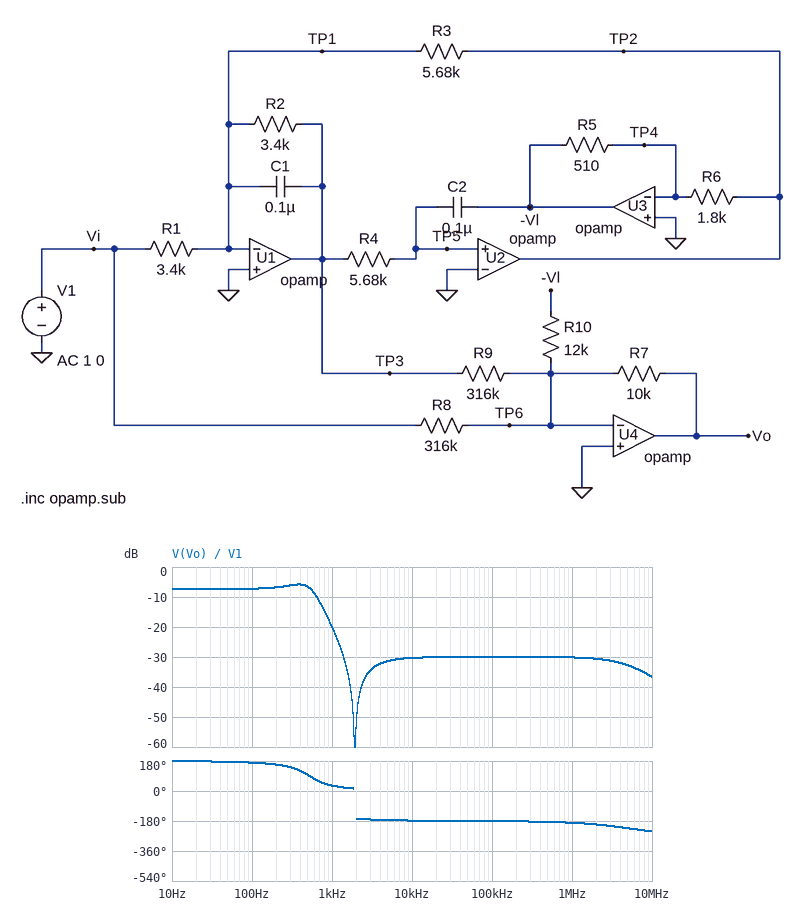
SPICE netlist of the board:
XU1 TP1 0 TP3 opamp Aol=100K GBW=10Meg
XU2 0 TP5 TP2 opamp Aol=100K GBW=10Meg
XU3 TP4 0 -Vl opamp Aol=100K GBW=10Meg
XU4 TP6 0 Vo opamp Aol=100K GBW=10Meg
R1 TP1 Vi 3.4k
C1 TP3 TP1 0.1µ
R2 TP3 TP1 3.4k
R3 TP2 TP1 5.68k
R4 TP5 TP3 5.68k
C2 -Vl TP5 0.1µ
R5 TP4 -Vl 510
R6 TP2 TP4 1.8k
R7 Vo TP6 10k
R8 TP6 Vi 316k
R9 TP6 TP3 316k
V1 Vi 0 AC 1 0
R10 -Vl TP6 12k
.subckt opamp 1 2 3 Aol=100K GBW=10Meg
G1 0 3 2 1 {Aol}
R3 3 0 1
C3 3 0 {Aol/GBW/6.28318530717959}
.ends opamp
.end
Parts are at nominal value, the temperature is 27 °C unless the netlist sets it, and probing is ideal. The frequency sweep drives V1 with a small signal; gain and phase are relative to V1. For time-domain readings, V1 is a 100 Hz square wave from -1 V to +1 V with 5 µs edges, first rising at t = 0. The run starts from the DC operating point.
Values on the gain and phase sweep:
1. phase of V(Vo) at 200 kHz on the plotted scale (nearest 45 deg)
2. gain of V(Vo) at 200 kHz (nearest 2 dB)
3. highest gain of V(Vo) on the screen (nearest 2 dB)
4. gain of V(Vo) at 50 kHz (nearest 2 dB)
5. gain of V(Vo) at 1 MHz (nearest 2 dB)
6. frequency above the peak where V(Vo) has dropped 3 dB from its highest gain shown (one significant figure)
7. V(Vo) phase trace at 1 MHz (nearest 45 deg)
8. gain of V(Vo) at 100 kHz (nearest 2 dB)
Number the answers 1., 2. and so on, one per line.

1. -180 deg
2. -30 dB
3. -6 dB
4. -30 dB
5. -30 dB
6. 600 Hz
7. -180 deg
8. -30 dB
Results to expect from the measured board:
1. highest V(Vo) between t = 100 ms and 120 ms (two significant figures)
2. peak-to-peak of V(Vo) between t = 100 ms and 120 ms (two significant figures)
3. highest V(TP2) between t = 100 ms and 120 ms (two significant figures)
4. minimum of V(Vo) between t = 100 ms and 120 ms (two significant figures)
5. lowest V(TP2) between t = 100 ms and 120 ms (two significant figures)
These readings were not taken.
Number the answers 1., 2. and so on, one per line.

1. 590 mV
2. 1.2 V
3. 2.4 V
4. -590 mV
5. -2.4 V
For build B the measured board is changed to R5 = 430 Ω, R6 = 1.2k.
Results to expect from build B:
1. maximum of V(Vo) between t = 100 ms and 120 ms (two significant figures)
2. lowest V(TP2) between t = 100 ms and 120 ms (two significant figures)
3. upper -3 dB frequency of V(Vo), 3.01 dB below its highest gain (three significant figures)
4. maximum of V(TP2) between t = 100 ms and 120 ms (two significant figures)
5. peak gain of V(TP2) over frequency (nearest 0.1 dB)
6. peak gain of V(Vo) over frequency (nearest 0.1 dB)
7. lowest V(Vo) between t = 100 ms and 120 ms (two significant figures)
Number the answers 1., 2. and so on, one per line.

1. 690 mV
2. -2.2 V
3. 529 Hz
4. 2.2 V
5. 5.7 dB
6. -4.5 dB
7. -690 mV
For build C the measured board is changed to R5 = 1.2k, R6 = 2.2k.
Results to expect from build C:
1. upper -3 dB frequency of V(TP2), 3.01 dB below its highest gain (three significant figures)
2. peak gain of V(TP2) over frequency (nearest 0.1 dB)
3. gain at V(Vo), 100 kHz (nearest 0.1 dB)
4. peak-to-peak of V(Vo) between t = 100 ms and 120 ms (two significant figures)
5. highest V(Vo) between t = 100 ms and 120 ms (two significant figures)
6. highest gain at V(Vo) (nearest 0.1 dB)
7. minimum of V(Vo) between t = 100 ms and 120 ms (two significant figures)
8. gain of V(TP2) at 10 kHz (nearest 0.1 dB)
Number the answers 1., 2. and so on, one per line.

1. 417 Hz
2. 4.7 dB
3. -30.0 dB
4. 1.8 V
5. 920 mV
6. -1.9 dB
7. -920 mV
8. -52.4 dB
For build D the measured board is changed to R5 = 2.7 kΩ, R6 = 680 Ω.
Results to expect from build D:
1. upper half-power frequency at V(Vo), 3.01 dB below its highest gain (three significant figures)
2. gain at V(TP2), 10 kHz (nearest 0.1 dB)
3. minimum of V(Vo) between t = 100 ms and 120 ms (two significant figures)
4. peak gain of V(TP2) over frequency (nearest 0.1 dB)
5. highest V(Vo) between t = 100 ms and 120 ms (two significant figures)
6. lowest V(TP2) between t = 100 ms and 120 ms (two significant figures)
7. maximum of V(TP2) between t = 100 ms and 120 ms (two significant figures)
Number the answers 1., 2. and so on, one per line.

1. 46.3 Hz
2. -69.6 dB
3. -3.2 V
4. 4.5 dB
5. 3.2 V
6. -980 mV
7. 980 mV
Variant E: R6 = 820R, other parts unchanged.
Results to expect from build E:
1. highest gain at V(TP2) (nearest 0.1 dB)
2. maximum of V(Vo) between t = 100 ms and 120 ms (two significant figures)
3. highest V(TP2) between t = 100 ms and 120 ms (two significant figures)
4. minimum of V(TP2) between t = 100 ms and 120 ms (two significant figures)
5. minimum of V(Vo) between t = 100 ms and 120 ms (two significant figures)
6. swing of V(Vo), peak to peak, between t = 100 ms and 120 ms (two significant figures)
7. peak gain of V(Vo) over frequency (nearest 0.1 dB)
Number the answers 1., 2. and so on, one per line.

1. 4.5 dB
2. 1.0 V
3. 1.9 V
4. -1.9 V
5. -1.0 V
6. 2.0 V
7. -0.9 dB
